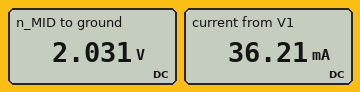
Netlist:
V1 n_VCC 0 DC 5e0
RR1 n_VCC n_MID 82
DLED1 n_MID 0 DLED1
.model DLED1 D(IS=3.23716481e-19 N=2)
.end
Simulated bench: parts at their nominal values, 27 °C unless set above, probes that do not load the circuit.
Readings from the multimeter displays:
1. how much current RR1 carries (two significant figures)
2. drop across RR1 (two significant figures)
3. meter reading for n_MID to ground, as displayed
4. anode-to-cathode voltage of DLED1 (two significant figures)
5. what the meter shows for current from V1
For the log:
36 mA
3.0 V
2.031 V
2.0 V
36.21 mA
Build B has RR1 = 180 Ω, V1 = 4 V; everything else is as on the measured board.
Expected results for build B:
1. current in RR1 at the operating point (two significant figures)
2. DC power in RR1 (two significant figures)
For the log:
11 mA
23 mW
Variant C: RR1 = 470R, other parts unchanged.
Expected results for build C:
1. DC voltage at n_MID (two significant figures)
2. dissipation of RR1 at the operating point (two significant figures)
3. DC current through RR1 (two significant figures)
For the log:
1.9 V
20 mW
6.5 mA
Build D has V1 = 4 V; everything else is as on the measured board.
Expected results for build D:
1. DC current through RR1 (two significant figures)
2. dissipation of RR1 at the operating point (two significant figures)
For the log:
24 mA
48 mW
